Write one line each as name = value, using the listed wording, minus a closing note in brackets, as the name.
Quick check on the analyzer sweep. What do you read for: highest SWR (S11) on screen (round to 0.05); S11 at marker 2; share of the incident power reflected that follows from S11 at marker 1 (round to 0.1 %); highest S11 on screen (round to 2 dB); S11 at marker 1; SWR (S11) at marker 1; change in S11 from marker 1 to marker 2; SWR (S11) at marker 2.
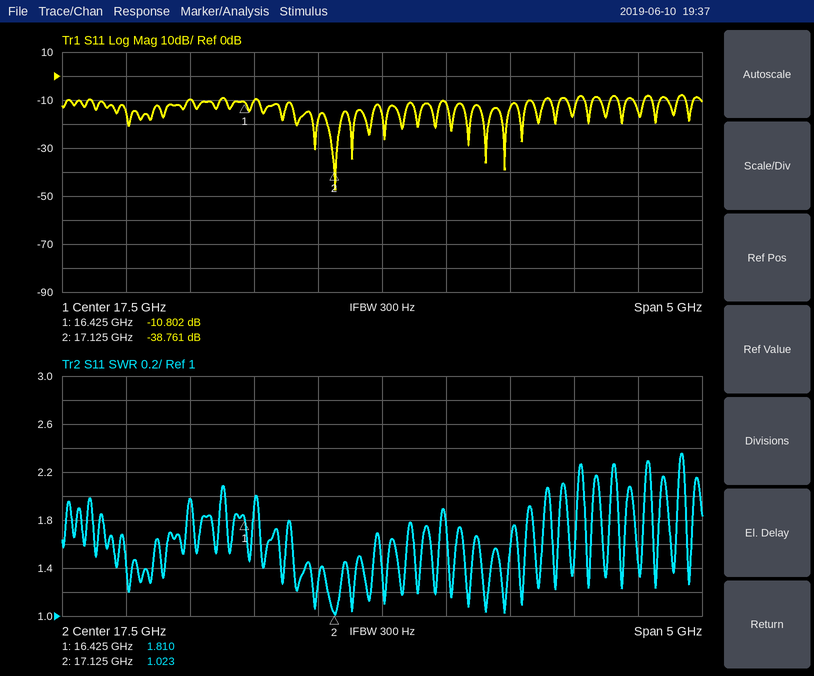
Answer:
highest SWR (S11) on screen = 2.35
S11 at marker 2 = -38.761 dB
share of the incident power reflected that follows from S11 at marker 1 = 8.3 %
highest S11 on screen = -8 dB
S11 at marker 1 = -10.802 dB
SWR (S11) at marker 1 = 1.810
change in S11 from marker 1 to marker 2 = -27.959 dB
SWR (S11) at marker 2 = 1.023
